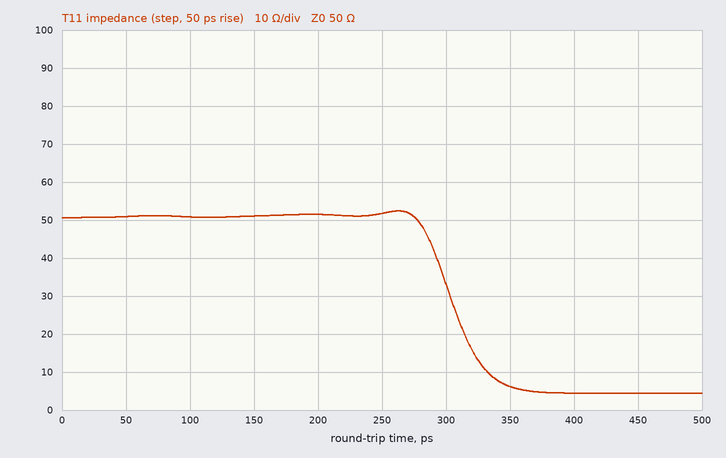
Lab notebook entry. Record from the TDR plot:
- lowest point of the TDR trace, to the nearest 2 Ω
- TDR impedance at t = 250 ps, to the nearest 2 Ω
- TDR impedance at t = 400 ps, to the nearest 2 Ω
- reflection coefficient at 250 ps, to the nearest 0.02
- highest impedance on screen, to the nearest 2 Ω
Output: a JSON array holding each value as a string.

["4 Ω", "52 Ω", "4 Ω", "+0.02", "52 Ω"]
